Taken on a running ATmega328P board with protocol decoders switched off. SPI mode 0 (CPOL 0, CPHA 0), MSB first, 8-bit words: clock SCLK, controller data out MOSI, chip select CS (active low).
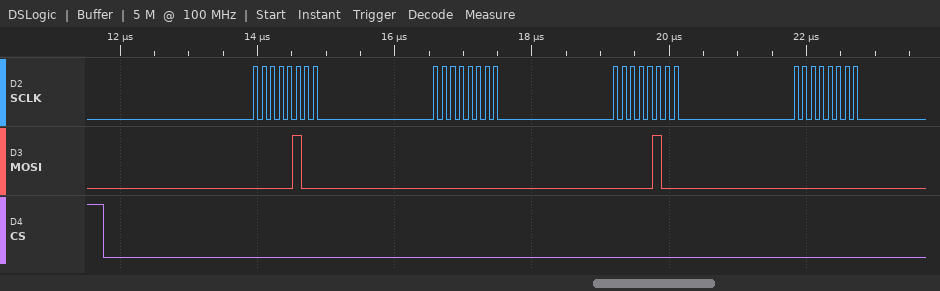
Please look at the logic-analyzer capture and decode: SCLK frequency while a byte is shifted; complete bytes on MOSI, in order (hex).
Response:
8 MHz
04 00 04 00
